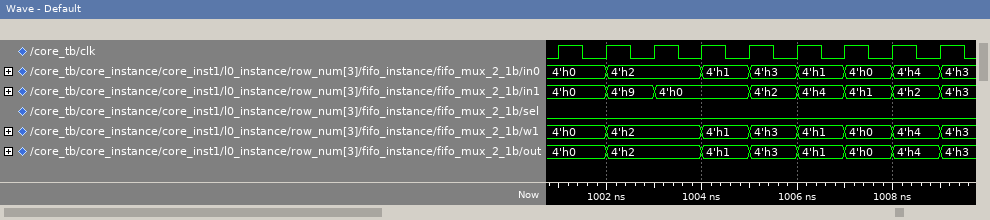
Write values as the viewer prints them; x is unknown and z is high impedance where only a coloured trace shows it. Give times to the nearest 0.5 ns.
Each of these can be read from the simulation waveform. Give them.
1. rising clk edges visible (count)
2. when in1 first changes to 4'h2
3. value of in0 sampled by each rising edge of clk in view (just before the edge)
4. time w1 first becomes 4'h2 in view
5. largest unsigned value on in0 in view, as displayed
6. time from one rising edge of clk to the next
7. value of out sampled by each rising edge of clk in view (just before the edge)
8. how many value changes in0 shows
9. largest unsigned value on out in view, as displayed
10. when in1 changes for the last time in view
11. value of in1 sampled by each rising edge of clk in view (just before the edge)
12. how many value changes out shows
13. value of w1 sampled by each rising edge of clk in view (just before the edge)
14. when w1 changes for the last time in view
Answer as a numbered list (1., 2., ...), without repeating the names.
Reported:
1. 9
2. 1005 ns
3. 4'h0, 4'h0, 4'h2, 4'h2, 4'h1, 4'h3, 4'h1, 4'h0, 4'h4
4. 1002 ns
5. 4'h4
6. 1 ns
7. 4'h0, 4'h0, 4'h2, 4'h2, 4'h1, 4'h3, 4'h1, 4'h0, 4'h4
8. 7
9. 4'h4
10. 1009 ns
11. 4'h0, 4'h0, 4'h9, 4'h0, 4'h0, 4'h2, 4'h4, 4'h1, 4'h2
12. 7
13. 4'h0, 4'h0, 4'h2, 4'h2, 4'h1, 4'h3, 4'h1, 4'h0, 4'h4
14. 1009 ns
